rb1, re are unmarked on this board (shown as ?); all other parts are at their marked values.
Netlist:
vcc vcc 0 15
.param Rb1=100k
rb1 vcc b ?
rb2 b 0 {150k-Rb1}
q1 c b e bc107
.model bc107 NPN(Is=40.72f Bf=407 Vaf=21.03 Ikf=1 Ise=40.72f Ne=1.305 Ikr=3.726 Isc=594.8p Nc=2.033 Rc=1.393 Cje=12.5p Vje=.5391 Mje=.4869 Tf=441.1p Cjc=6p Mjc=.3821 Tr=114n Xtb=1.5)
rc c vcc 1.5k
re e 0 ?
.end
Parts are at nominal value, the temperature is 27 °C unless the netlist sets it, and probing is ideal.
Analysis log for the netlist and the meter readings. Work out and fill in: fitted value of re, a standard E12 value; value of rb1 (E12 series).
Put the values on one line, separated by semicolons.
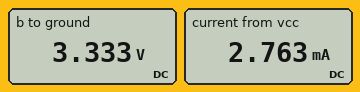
1 kΩ; 150 kΩ
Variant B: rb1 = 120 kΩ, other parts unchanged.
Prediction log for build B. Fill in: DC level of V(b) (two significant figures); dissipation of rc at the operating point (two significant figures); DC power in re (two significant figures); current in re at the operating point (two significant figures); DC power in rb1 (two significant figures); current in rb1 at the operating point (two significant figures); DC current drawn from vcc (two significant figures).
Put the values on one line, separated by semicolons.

3.9 V; 16 mW; 11 mW; 3.3 mA; 1.0 mW; 92 µA; 3.4 mA
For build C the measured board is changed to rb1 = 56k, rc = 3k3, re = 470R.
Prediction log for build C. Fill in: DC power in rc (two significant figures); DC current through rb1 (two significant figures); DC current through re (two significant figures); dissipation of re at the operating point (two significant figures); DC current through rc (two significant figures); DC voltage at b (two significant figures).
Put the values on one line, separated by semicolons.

51 mW; 220 µA; 4.1 mA; 7.9 mW; 3.9 mA; 2.6 V
